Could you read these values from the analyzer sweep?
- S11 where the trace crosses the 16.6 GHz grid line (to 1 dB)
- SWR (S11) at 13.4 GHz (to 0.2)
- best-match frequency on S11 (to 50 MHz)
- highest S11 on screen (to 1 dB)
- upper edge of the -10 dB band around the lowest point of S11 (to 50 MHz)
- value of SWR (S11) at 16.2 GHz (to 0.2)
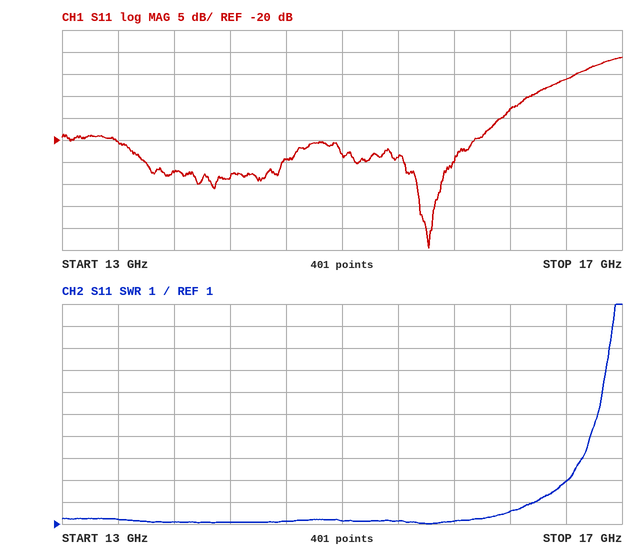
-6 dB
1.2
15.60 GHz
-1 dB
16.35 GHz
1.6
